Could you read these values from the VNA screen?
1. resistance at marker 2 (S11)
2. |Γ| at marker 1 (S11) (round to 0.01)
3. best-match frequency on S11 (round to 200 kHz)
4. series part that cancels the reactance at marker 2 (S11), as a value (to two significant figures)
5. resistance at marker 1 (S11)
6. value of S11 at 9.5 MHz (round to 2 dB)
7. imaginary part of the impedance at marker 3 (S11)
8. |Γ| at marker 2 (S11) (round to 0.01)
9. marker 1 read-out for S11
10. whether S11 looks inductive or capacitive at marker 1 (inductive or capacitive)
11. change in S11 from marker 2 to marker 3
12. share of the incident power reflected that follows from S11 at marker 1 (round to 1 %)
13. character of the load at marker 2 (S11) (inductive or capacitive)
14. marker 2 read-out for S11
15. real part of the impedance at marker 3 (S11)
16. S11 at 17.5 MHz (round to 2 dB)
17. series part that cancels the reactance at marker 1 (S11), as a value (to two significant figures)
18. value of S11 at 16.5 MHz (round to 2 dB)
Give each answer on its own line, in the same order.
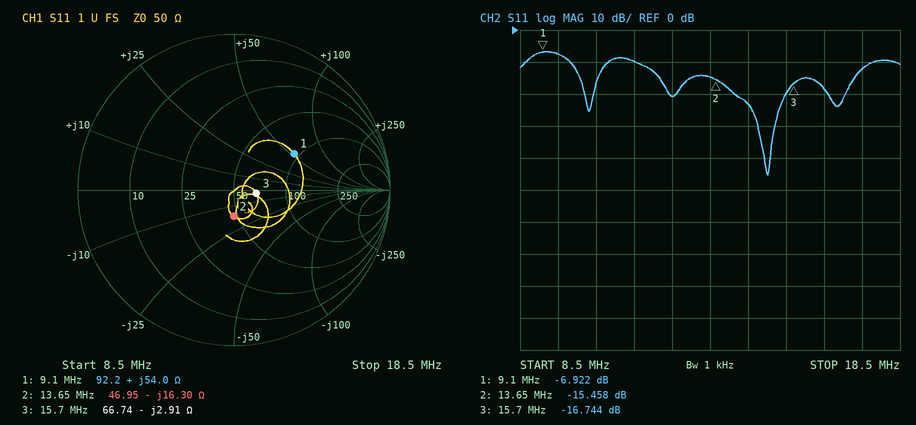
46.95 Ω
0.45
15.0 MHz
190 nH
92.2 Ω
-8 dB
-2.91 Ω
0.17
-6.922 dB
inductive
-1.286 dB
20 %
capacitive
-15.458 dB
66.74 Ω
-12 dB
320 pF
-18 dB
